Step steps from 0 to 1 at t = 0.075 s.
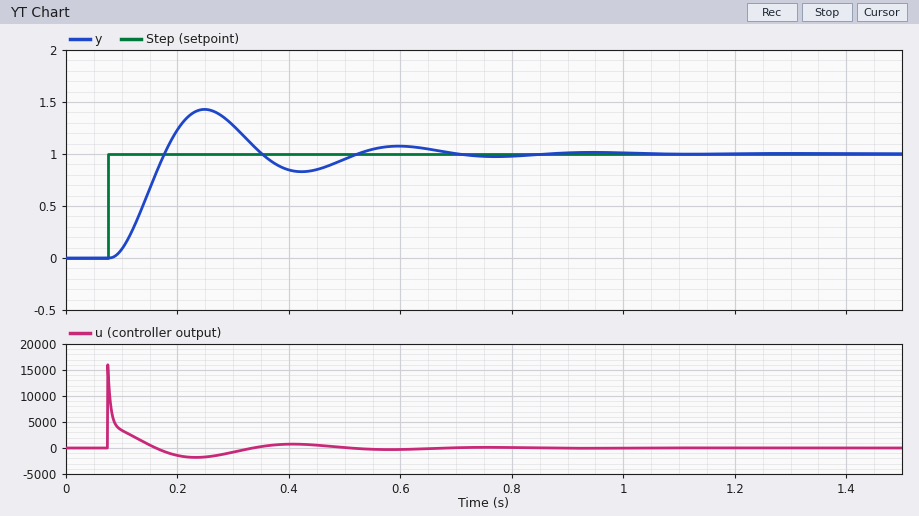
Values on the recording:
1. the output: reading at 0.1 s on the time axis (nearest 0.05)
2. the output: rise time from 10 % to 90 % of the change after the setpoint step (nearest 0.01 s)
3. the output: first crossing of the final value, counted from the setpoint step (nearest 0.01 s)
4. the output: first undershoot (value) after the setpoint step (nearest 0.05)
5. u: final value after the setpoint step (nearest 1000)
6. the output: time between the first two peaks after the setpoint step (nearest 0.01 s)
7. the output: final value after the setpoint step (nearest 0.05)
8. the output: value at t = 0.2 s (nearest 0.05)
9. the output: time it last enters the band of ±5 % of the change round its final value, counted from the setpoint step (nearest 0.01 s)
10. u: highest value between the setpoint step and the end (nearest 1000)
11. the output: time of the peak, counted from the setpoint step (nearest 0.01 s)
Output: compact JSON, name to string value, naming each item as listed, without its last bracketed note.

{"the output: reading at 0.1 s on the time axis": "0.10", "the output: rise time from 10 % to 90 % of the change after the setpoint step": "0.07 s", "the output: first crossing of the final value, counted from the setpoint step": "0.10 s", "the output: first undershoot (value) after the setpoint step": "0.85", "u: final value after the setpoint step": "0", "the output: time between the first two peaks after the setpoint step": "0.35 s", "the output: final value after the setpoint step": "1.00", "the output: value at t = 0.2 s": "1.25", "the output: time it last enters the band of ±5 % of the change round its final value, counted from the setpoint step": "0.57 s", "u: highest value between the setpoint step and the end": "16000", "the output: time of the peak, counted from the setpoint step": "0.17 s"}
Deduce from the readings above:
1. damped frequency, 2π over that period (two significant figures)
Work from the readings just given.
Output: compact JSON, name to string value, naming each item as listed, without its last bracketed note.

{"damped frequency, 2π over that period": "18 rad/s"}
